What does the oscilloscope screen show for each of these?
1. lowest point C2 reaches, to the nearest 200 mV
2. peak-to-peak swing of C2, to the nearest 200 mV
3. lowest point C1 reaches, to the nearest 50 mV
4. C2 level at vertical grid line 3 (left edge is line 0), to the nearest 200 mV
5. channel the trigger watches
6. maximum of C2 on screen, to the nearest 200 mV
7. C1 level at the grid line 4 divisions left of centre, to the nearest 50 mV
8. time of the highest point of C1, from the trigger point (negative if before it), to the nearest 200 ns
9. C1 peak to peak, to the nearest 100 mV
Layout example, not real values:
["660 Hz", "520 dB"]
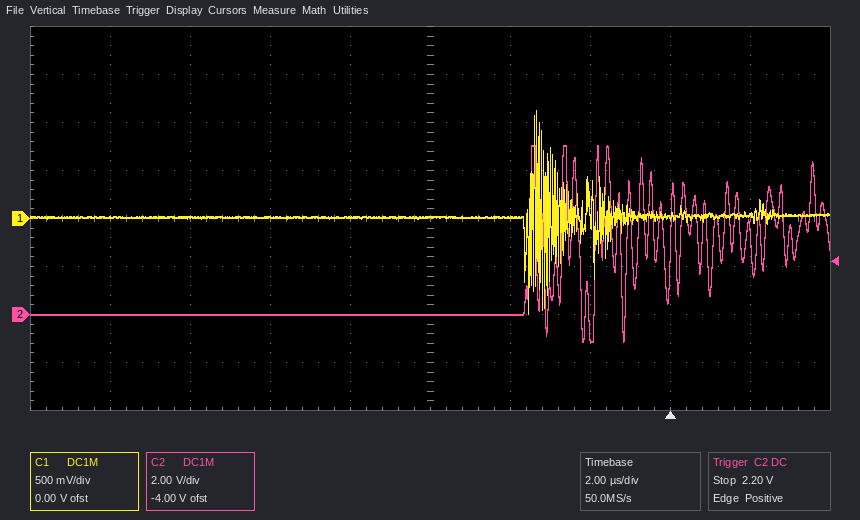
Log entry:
["-1.2 V", "8.2 V", "-1.00 V", "0.0 V", "C2", "7.0 V", "0 mV", "-3.4 µs", "2.10 V"]
